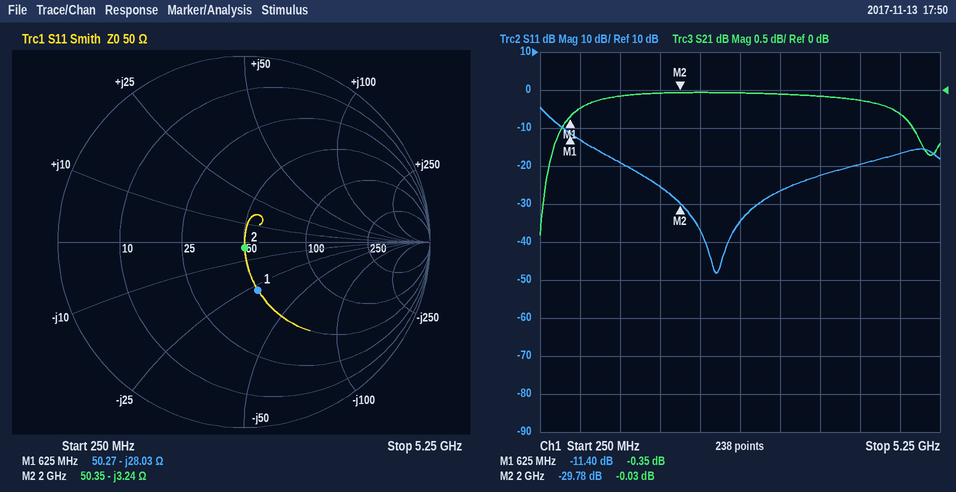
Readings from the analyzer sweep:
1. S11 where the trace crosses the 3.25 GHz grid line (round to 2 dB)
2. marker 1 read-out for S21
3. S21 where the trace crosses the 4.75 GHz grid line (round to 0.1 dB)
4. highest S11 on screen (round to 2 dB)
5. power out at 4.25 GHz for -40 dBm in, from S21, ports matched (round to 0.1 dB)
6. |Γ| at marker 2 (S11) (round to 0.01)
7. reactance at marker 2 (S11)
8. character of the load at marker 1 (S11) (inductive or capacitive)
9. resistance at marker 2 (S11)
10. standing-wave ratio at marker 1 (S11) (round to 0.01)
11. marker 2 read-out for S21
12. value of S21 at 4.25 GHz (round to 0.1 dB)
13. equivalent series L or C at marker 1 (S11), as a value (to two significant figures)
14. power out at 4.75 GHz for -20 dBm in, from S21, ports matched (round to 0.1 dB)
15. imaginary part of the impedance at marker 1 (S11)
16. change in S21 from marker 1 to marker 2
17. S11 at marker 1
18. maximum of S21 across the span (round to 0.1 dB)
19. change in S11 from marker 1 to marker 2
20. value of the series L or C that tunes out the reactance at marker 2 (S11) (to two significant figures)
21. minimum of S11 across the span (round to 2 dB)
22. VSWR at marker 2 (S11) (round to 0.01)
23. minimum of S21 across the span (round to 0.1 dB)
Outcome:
-26 dB
-0.35 dB
-0.3 dB
-4 dB
-40.1 dBm
0.03
-3.24 Ω
capacitive
50.35 Ω
1.74
-0.03 dB
-0.1 dB
9.1 pF
-20.3 dBm
-28.03 Ω
0.32 dB
-11.40 dB
0.0 dB
-18.38 dB
260 pH
-48 dB
1.07
-1.9 dB
